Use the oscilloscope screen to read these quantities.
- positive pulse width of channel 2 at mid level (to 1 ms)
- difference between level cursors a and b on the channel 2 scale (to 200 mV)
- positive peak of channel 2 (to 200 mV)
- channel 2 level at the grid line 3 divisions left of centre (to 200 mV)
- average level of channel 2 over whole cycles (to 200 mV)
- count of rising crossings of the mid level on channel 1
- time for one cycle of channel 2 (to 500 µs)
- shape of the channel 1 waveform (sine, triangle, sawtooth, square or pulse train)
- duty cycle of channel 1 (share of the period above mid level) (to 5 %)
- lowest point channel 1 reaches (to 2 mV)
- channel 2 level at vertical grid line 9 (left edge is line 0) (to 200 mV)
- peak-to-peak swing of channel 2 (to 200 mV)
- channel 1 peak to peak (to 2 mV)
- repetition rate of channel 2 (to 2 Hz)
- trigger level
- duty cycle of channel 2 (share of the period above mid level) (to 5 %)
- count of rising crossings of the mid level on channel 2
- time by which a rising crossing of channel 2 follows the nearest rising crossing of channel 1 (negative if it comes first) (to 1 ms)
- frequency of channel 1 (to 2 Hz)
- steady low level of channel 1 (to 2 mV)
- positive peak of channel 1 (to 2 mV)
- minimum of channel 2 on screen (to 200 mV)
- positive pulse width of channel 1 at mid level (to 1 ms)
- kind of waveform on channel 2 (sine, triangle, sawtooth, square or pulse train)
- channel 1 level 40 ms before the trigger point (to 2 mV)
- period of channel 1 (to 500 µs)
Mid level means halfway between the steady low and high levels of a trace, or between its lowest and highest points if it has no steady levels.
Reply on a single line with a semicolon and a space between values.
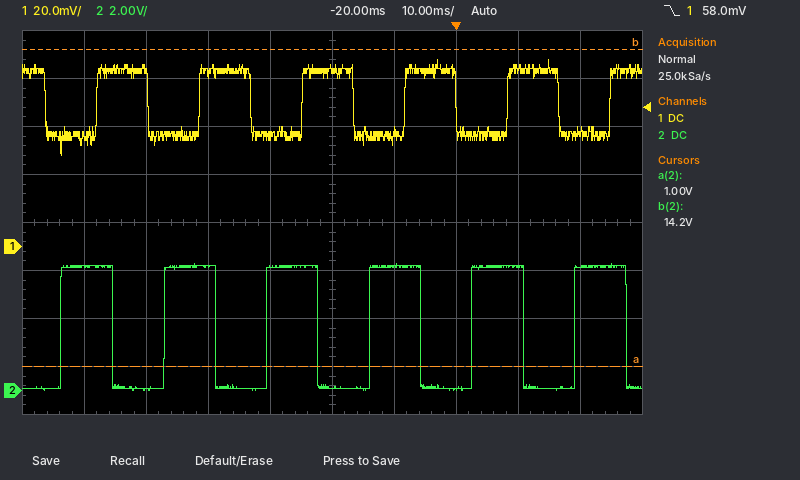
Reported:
8 ms; 13.2 V; 5.2 V; 0.0 V; 2.6 V; 6; 16.5 ms; square; 50 %; 38 mV; 5.2 V; 5.2 V; 40 mV; 60 Hz; 58.0 mV; 50 %; 6; -6 ms; 60 Hz; 46 mV; 78 mV; 0.0 V; 8 ms; square; 72 mV; 16.5 ms
